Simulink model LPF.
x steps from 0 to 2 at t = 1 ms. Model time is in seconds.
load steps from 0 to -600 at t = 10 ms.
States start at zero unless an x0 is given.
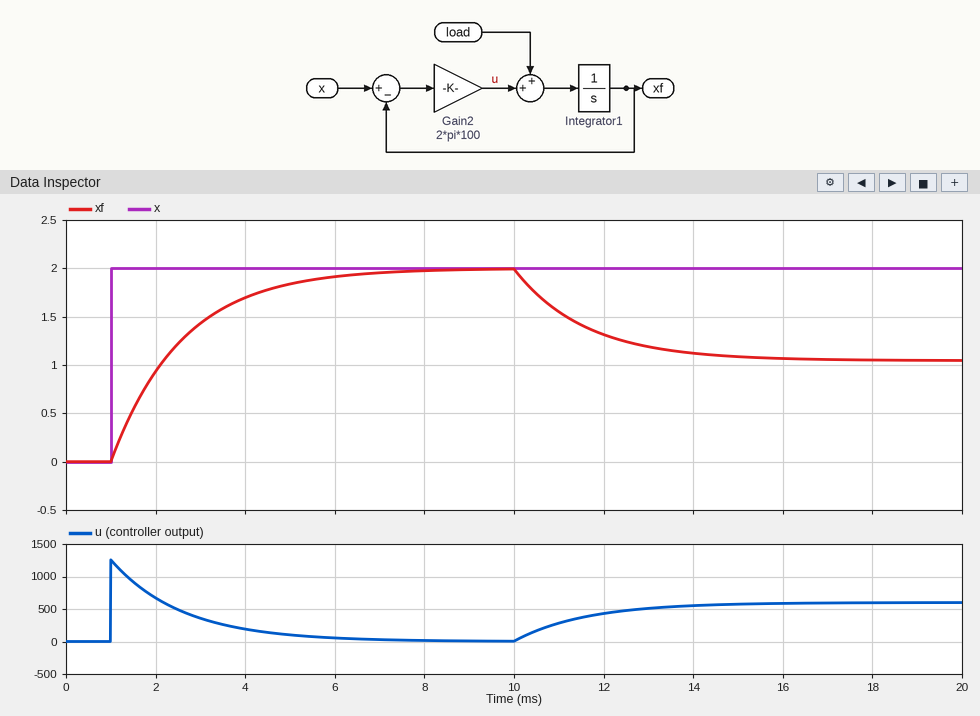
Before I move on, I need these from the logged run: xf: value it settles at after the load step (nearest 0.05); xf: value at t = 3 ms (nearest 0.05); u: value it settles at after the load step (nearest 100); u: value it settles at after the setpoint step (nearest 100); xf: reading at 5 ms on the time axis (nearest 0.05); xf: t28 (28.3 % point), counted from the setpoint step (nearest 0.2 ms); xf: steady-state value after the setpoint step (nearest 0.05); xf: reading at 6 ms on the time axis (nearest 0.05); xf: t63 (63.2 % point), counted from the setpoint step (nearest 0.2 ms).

1.05
1.45
600
0
1.85
0.6 ms
2.00
1.90
1.6 ms
